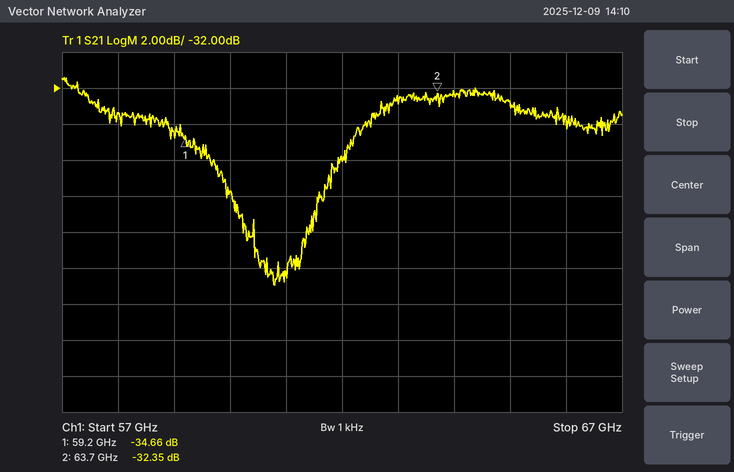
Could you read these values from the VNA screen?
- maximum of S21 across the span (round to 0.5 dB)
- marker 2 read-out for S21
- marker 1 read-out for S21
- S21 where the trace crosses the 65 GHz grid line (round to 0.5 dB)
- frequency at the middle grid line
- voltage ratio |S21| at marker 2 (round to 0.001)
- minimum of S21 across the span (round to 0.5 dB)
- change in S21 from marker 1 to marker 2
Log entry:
-31.5 dB
-32.35 dB
-34.66 dB
-33.0 dB
62 GHz
0.024
-43.0 dB
2.31 dB
